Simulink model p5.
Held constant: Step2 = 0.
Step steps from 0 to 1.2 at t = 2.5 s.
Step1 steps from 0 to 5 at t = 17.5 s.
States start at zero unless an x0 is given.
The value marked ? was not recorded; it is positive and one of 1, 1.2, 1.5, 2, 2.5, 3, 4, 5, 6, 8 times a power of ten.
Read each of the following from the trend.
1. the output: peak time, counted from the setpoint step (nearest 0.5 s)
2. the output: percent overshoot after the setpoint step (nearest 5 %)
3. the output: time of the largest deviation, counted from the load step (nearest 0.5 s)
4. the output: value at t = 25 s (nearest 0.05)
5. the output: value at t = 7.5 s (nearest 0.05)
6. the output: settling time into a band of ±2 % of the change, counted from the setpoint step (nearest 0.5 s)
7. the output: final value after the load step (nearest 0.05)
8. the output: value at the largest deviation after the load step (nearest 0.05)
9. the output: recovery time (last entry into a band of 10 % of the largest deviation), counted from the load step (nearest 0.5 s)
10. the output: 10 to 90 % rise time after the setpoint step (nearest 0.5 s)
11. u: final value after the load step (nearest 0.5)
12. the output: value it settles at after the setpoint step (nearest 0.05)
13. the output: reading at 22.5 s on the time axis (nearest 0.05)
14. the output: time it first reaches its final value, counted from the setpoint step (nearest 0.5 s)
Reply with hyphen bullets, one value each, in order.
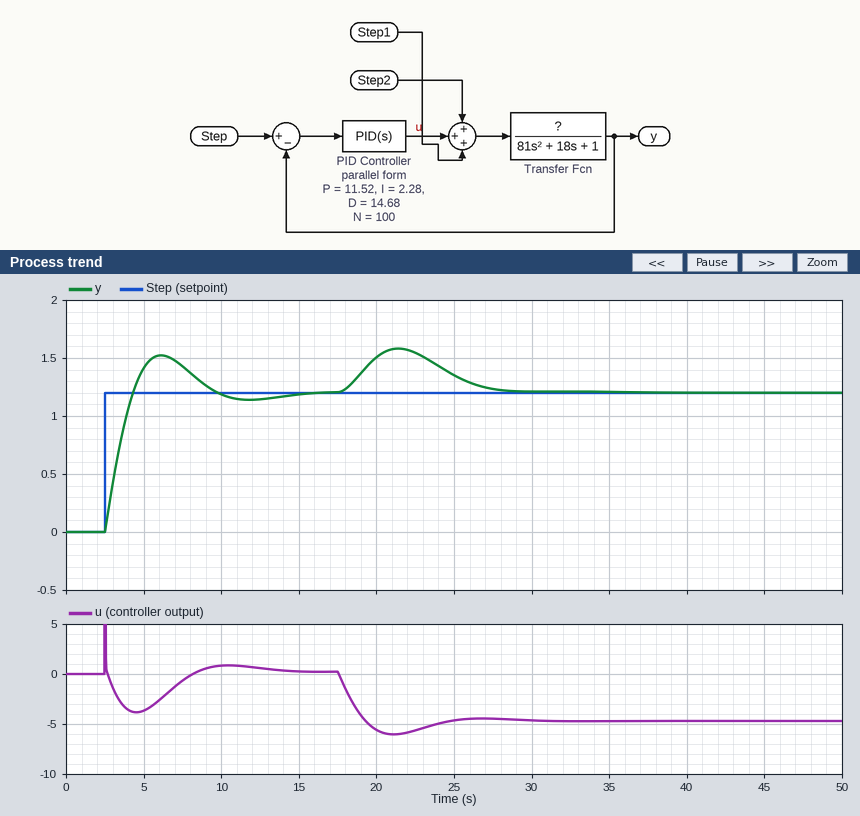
- 3.5 s
- 25 %
- 4.0 s
- 1.35
- 1.45
- 12.0 s
- 1.20
- 1.60
- 10.0 s
- 1.5 s
- -4.5
- 1.20
- 1.55
- 2.0 s
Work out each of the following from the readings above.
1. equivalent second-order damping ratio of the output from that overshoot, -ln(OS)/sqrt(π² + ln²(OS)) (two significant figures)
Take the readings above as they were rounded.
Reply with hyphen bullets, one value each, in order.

- 0.40
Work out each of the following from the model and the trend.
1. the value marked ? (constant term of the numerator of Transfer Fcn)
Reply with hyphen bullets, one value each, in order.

- 4
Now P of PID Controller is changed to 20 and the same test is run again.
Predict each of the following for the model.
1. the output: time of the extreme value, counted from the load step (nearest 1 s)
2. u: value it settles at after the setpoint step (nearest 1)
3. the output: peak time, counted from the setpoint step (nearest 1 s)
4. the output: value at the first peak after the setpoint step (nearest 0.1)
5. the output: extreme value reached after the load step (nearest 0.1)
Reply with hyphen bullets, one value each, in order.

- 3 s
- 0
- 3 s
- 1.6
- 1.5
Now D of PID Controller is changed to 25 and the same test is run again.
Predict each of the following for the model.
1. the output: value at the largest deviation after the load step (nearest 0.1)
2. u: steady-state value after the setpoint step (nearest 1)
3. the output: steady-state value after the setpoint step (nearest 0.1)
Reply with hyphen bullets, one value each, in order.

- 1.5
- 0
- 1.2
